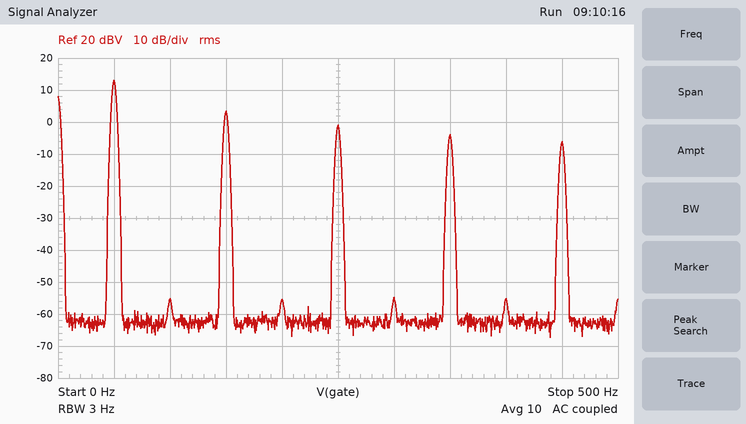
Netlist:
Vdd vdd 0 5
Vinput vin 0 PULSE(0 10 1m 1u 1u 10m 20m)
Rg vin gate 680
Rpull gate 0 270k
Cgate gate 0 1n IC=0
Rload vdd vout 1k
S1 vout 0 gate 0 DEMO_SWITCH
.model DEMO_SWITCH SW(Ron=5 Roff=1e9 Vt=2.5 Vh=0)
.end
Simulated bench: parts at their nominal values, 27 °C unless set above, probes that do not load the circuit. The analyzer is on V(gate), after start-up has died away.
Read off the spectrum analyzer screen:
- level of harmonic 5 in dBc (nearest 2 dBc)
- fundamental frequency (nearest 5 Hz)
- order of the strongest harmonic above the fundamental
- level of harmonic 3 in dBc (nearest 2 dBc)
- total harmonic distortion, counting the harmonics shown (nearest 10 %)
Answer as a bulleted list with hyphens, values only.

- -14 dBc
- 50 Hz
- 3
- -10 dBc
- 40 %
